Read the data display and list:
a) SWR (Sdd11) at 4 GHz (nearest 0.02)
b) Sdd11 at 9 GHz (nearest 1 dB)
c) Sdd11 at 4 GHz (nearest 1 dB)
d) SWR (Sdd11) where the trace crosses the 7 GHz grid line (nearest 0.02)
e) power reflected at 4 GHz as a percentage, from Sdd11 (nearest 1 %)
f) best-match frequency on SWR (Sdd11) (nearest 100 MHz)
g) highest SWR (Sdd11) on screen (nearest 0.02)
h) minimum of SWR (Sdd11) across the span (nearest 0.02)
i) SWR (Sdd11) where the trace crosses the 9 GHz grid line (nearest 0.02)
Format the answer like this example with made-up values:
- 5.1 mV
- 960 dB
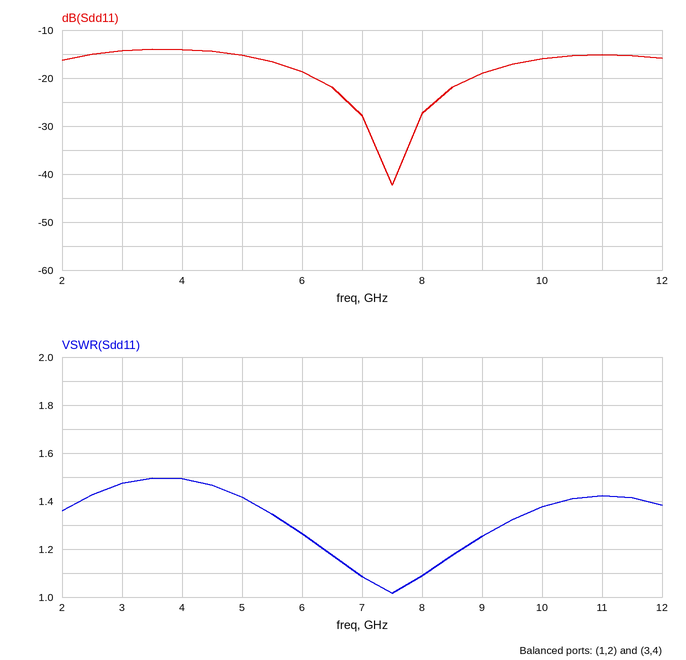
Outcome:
- 1.50
- -19 dB
- -14 dB
- 1.08
- 4 %
- 7.5 GHz
- 1.50
- 1.02
- 1.26
